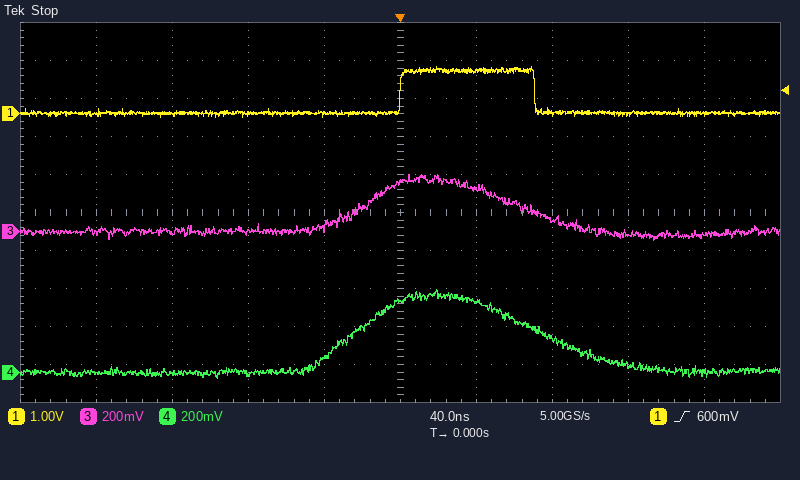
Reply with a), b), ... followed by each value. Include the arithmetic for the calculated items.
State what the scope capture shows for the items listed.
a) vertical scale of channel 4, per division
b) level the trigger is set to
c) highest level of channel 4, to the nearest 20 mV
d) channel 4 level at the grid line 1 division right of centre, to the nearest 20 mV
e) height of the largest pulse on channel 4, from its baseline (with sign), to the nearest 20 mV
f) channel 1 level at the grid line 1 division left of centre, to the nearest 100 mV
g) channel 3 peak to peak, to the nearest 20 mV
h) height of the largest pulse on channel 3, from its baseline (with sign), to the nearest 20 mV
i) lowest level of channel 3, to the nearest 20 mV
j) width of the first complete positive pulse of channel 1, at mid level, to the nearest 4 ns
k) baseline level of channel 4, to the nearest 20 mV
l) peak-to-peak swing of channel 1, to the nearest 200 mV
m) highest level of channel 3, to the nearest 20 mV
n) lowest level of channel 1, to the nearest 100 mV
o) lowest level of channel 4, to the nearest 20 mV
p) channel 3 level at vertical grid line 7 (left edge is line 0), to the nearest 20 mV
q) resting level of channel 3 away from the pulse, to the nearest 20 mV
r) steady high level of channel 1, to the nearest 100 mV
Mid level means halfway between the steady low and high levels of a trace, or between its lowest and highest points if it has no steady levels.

a) 200 mV
b) 600 mV
c) 440 mV
d) 380 mV
e) 440 mV − (0 mV) = +440 mV
f) 0.0 V
g) 300 mV − (-40 mV) = 340 mV
h) 300 mV − (0 mV) = +300 mV
i) -40 mV
j) 72 ns
k) 0 mV
l) 1.4 V
m) 300 mV
n) -100 mV
o) -40 mV
p) 60 mV
q) 0 mV
r) 1.1 V
